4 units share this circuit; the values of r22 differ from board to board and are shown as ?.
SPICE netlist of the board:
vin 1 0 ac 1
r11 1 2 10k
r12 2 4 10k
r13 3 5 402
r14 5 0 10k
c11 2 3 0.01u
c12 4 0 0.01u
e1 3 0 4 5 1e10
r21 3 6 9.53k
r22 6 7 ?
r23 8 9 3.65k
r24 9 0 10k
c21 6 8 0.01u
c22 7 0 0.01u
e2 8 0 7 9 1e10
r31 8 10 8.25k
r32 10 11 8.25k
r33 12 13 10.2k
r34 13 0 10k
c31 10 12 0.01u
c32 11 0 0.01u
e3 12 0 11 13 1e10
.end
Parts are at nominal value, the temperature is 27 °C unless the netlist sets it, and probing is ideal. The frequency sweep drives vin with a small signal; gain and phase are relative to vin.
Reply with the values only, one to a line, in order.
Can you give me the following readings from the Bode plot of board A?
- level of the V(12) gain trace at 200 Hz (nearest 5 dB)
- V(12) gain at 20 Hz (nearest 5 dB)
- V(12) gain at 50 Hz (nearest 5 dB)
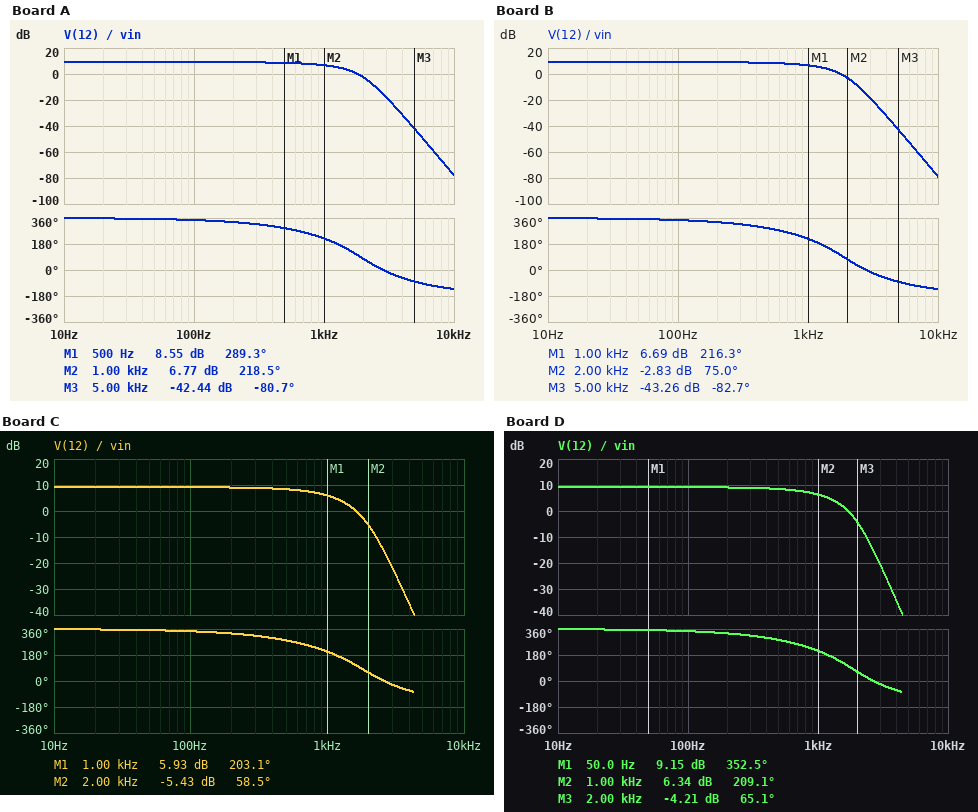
10 dB
10 dB
10 dB
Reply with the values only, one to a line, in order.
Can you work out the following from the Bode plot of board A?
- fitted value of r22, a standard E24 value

5.6 kΩ
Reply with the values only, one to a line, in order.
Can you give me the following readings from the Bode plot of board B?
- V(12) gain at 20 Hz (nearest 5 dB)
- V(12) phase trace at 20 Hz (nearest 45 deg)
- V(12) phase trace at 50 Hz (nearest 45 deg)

10 dB
360 deg
360 deg
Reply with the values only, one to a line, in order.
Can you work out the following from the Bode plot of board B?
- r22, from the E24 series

6.2 kΩ
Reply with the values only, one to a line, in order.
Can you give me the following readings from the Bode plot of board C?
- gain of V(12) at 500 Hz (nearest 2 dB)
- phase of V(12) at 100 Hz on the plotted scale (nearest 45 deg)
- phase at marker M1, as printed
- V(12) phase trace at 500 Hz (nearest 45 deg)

8 dB
360 deg
203.1 deg
270 deg
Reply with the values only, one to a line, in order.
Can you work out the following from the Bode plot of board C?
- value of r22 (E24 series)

10 kΩ
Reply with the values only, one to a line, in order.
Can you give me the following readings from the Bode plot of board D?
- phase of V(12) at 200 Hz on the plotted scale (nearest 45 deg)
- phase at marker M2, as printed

315 deg
209.1 deg
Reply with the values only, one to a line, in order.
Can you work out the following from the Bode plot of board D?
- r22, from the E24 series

8.2 kΩ
